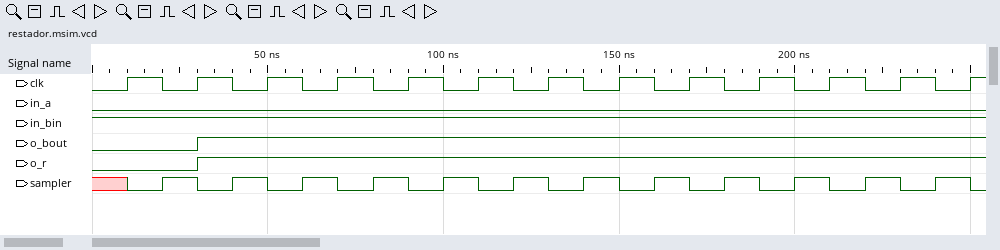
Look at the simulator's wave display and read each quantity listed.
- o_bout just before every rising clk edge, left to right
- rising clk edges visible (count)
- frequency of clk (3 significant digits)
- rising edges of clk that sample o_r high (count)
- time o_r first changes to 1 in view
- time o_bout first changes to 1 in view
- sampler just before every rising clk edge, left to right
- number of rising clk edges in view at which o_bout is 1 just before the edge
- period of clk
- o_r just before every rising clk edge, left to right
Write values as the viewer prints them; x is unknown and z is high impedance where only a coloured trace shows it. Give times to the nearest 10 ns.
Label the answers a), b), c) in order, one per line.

a) 0 0 1 1 1 1 1 1 1 1 1 1 1
b) 13
c) 50.0 MHz
d) 11
e) 30 ns
f) 30 ns
g) x 1 1 1 1 1 1 1 1 1 1 1 1
h) 11
i) 20 ns
j) 0 0 1 1 1 1 1 1 1 1 1 1 1
